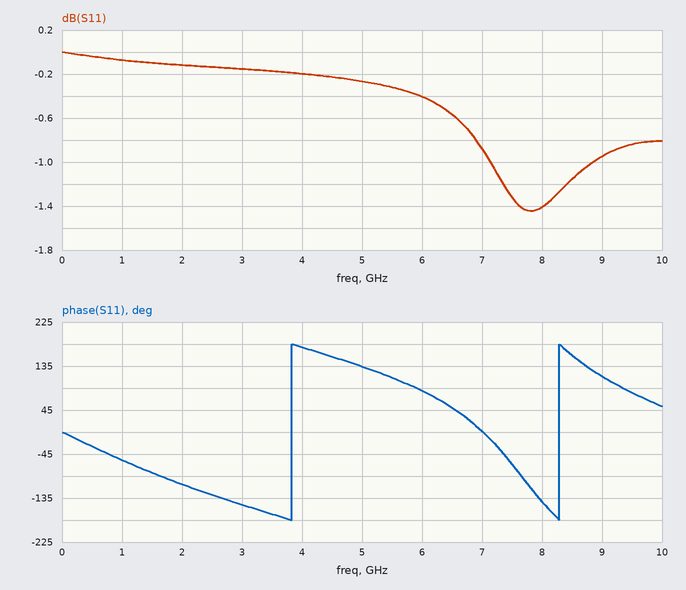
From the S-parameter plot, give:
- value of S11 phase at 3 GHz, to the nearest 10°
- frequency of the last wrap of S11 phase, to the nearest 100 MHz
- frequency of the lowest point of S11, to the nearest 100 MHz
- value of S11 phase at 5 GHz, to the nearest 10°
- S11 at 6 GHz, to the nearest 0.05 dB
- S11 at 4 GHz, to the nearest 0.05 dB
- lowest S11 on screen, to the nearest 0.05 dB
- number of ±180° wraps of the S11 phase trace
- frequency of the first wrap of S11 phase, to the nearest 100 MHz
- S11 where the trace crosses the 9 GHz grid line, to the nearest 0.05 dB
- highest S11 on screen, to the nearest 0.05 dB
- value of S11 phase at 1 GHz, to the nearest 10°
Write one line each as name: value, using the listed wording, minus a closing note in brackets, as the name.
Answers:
value of S11 phase at 3 GHz, to the nearest 10°: -150°
frequency of the last wrap of S11 phase, to the nearest 100 MHz: 8.3 GHz
frequency of the lowest point of S11, to the nearest 100 MHz: 7.8 GHz
value of S11 phase at 5 GHz, to the nearest 10°: 130°
S11 at 6 GHz, to the nearest 0.05 dB: -0.40 dB
S11 at 4 GHz, to the nearest 0.05 dB: -0.20 dB
lowest S11 on screen, to the nearest 0.05 dB: -1.45 dB
number of ±180° wraps of the S11 phase trace: 2
frequency of the first wrap of S11 phase, to the nearest 100 MHz: 3.8 GHz
S11 where the trace crosses the 9 GHz grid line, to the nearest 0.05 dB: -0.95 dB
highest S11 on screen, to the nearest 0.05 dB: 0.00 dB
value of S11 phase at 1 GHz, to the nearest 10°: -60°
